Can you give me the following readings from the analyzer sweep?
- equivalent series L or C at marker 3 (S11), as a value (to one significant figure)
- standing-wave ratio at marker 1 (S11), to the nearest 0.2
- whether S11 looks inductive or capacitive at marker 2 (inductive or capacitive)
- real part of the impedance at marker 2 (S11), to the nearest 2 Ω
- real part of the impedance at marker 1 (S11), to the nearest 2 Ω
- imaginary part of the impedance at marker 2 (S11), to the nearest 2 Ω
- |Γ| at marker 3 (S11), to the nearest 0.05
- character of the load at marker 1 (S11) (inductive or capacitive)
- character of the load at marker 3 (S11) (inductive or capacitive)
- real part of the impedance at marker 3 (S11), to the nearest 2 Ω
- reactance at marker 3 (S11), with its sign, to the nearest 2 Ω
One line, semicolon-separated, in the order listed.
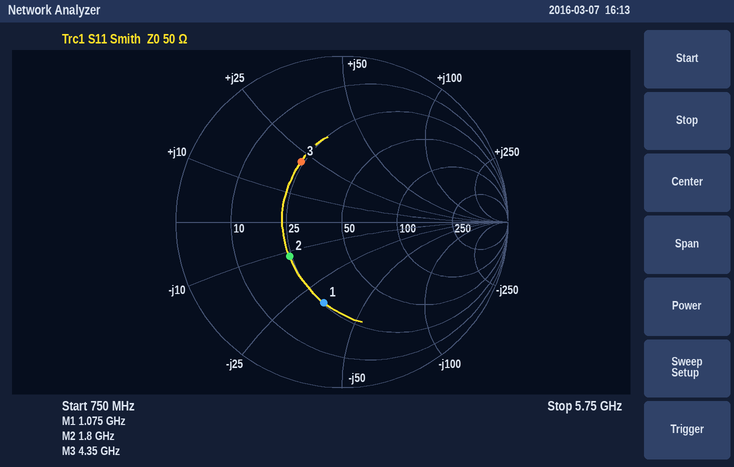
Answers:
800 pH; 3.0; capacitive; 24 Ω; 26 Ω; -12 Ω; 0.45; capacitive; inductive; 24 Ω; +22 Ω
